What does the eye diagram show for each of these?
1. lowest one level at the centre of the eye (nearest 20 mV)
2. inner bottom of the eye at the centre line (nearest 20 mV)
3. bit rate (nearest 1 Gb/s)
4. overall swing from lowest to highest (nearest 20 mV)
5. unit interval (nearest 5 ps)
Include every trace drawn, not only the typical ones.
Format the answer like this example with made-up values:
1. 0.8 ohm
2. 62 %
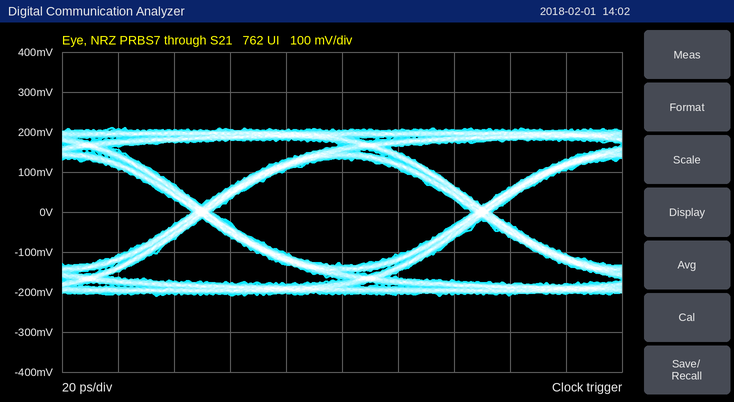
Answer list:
1. 140 mV
2. -140 mV
3. 10 Gb/s
4. 420 mV
5. 100 ps
